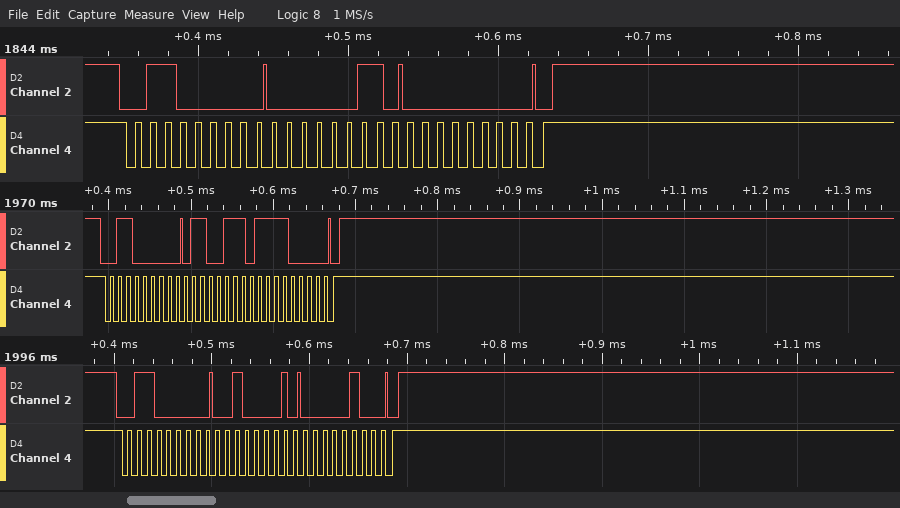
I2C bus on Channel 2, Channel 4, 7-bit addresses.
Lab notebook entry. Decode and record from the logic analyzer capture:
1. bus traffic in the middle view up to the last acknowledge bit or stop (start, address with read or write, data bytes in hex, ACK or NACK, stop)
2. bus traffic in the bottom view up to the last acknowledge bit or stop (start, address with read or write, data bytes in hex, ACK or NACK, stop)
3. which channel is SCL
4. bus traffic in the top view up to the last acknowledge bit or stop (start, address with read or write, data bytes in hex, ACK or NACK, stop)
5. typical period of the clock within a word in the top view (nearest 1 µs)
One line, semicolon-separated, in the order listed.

start, address 30 write ACK, 67 ACK, F0 ACK, stop; start, address 30 write ACK, 21 ACK, 04 ACK, stop; Channel 4; start, address 30 write ACK, 03 ACK, 00 ACK, stop; 10 µs
